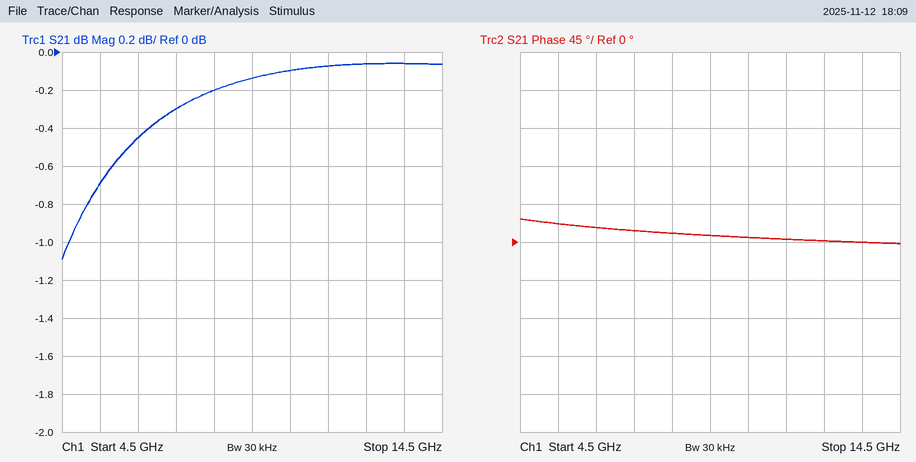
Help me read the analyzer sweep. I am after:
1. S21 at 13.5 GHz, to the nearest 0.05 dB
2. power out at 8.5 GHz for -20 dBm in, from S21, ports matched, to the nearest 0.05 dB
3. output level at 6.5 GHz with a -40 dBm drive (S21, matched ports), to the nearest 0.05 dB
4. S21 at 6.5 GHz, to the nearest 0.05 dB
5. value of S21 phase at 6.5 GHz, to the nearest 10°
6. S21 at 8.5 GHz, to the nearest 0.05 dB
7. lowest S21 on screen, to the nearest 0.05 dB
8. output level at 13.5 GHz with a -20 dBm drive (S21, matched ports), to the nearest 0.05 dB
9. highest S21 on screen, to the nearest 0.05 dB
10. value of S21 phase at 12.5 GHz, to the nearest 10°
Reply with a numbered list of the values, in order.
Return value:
1. -0.05 dB
2. -20.20 dBm
3. -40.45 dBm
4. -0.45 dB
5. 20°
6. -0.20 dB
7. -1.10 dB
8. -20.05 dBm
9. -0.05 dB
10. 0°
